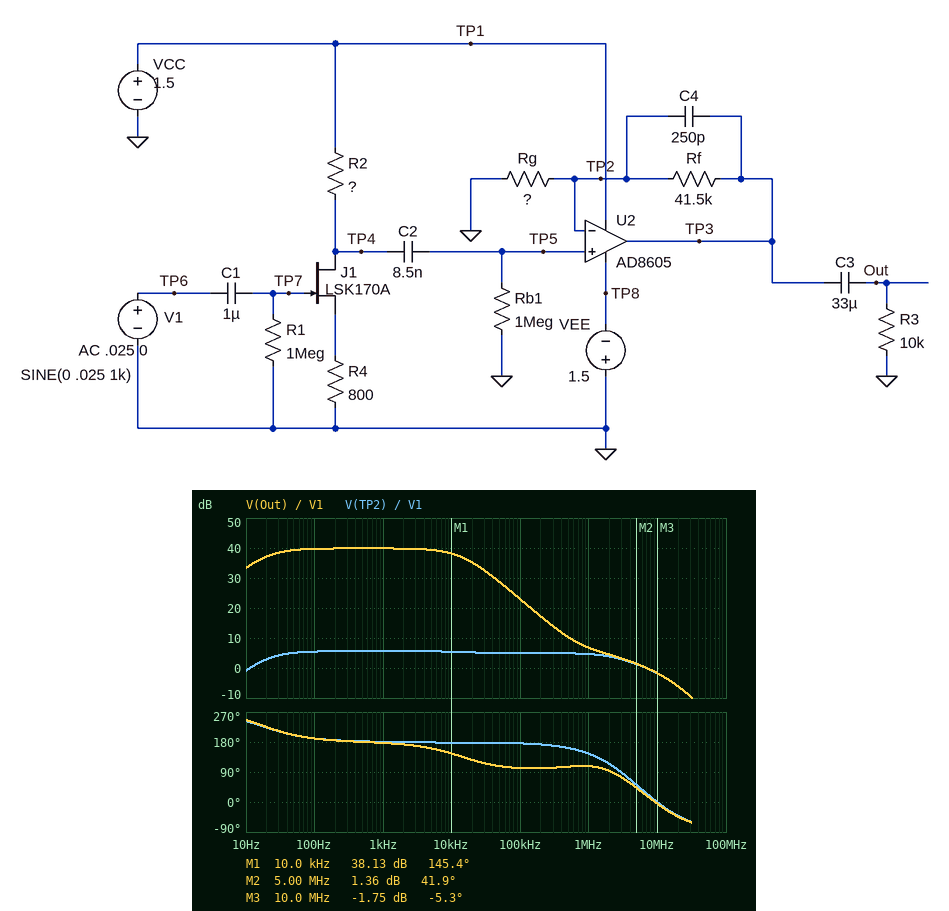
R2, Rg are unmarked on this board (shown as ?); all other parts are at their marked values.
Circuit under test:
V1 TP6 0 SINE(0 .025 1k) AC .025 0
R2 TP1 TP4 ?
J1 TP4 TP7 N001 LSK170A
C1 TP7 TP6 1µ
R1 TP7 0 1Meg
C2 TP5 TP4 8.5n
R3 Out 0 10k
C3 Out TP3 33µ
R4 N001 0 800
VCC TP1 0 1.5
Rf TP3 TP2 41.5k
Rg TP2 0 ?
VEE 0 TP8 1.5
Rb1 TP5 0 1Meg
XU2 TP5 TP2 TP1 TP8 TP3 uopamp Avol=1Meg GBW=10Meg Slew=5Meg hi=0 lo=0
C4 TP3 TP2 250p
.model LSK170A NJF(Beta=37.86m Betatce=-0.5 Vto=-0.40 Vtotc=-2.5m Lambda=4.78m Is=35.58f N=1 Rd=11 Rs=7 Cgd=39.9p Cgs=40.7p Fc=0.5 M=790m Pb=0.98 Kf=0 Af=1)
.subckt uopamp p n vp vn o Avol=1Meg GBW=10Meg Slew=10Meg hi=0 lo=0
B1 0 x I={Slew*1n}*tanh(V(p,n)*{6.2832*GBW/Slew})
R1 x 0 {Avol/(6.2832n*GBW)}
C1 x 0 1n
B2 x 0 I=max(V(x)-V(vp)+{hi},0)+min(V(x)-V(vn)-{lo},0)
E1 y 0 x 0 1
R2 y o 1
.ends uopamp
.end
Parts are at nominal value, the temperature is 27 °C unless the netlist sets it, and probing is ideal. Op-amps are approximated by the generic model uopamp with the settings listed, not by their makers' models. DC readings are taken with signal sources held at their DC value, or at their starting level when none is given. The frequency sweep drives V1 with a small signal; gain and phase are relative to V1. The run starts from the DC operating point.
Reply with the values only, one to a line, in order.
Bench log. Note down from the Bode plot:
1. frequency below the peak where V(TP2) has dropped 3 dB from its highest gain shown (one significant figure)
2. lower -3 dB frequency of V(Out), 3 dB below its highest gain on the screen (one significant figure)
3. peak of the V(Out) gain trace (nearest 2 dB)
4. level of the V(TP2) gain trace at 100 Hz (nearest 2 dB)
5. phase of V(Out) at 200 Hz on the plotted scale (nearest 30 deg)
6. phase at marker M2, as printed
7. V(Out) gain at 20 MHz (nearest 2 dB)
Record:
20 Hz
20 Hz
40 dB
6 dB
180 deg
41.9 deg
-6 dB
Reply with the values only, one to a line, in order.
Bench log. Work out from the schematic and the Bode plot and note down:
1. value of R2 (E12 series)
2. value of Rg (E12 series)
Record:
1.8 kΩ
820 Ω
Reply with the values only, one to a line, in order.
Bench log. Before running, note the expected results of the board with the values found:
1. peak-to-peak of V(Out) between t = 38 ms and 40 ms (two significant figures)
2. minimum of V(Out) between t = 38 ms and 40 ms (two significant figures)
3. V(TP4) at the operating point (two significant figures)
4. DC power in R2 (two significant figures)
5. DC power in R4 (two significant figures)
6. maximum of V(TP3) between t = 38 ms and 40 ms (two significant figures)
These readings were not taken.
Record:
3.0 V
-1.5 V
830 mV
250 µW
110 µW
1.5 V
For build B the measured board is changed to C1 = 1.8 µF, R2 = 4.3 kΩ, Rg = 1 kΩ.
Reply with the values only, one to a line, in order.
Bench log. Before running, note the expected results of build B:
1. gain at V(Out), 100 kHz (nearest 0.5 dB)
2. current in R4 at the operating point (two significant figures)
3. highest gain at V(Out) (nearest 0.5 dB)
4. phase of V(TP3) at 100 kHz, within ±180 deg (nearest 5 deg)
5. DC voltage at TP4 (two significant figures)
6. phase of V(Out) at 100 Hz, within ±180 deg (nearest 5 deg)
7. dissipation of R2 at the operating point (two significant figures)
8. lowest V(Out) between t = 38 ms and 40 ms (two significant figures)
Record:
-1.0 dB
290 µA
15.5 dB
90 deg
260 mV
-170 deg
360 µW
-140 mV
